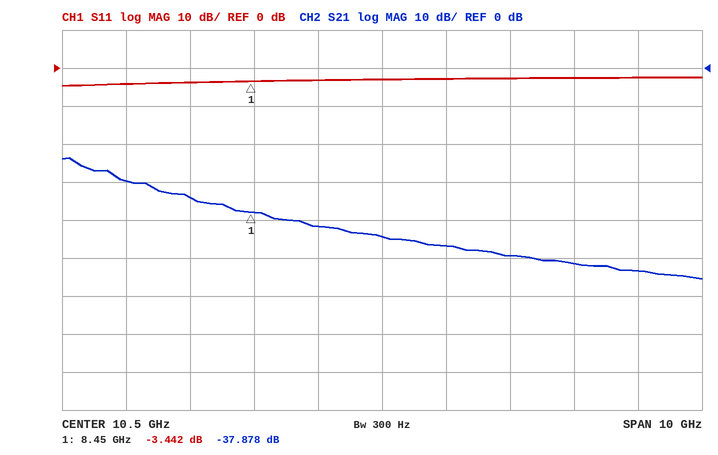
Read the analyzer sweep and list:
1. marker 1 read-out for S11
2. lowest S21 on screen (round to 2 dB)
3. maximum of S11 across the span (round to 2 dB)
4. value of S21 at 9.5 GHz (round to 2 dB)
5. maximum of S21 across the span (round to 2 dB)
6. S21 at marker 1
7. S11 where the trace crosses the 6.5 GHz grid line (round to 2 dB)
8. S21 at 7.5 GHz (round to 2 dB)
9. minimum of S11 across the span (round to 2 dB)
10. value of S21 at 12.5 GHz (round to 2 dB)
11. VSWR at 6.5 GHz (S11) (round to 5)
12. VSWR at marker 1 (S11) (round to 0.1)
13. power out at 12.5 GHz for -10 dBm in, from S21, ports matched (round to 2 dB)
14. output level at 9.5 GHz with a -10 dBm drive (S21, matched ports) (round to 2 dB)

-3.442 dB
-56 dB
-2 dB
-42 dB
-24 dB
-37.878 dB
-4 dB
-34 dB
-4 dB
-50 dB
5
5.1
-60 dBm
-52 dBm
